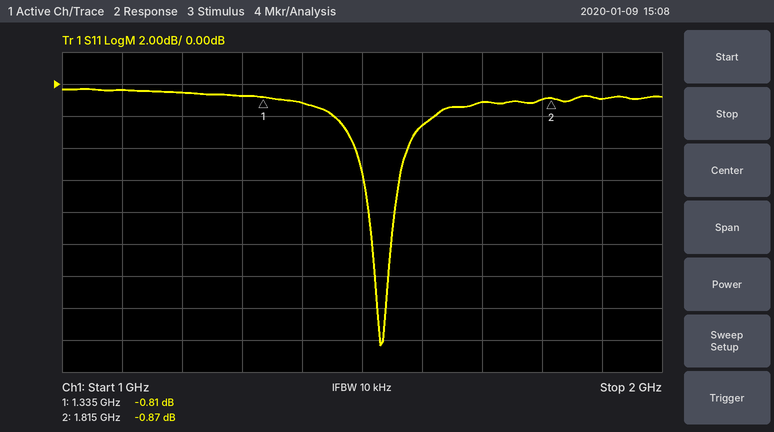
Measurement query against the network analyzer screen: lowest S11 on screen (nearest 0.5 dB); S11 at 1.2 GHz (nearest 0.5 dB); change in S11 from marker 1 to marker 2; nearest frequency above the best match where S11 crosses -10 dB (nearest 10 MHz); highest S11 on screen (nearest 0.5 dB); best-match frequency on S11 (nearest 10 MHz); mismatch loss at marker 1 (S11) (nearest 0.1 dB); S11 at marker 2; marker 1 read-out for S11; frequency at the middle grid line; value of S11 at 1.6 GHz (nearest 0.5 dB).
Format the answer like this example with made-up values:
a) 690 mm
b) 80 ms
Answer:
a) -16.5 dB
b) -0.5 dB
c) -0.06 dB
d) 1.55 GHz
e) -0.5 dB
f) 1.53 GHz
g) 7.7 dB
h) -0.87 dB
i) -0.81 dB
j) 1.5 GHz
k) -2.5 dB
